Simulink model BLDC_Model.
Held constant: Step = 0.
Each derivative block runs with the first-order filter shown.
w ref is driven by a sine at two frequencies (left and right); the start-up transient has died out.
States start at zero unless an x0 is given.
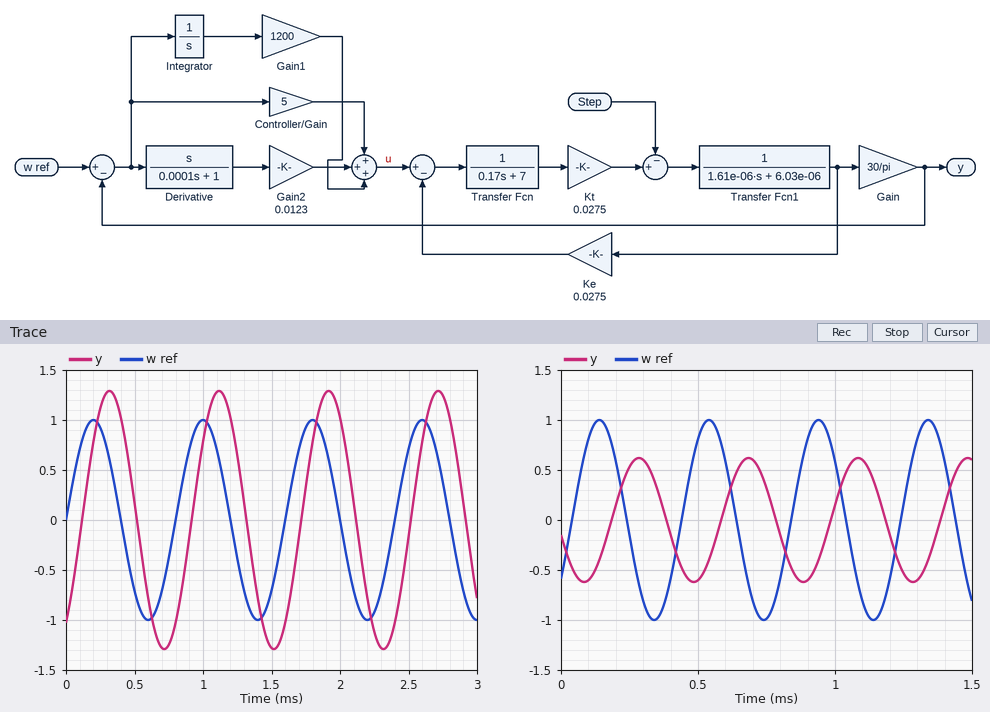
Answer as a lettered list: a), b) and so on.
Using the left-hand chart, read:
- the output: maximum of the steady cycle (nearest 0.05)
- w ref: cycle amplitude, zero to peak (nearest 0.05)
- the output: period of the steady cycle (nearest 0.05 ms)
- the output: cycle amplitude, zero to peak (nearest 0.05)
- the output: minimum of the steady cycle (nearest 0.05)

a) 1.30
b) 1.00
c) 0.80 ms
d) 1.30
e) -1.30
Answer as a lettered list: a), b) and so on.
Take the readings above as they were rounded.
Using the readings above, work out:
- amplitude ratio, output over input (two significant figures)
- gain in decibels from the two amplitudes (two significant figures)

a) 1.3
b) 2.3 dB
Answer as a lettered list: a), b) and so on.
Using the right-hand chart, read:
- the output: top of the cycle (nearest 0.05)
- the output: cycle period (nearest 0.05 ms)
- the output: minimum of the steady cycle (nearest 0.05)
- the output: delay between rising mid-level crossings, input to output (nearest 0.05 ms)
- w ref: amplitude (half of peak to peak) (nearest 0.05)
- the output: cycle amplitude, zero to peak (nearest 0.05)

a) 0.60
b) 0.40 ms
c) -0.60
d) 0.15 ms
e) 1.00
f) 0.60
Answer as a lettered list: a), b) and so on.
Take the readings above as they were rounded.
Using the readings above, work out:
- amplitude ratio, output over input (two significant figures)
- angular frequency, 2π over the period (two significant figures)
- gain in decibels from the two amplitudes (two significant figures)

a) 0.60
b) 16 rad/ms
c) -4.4 dB
